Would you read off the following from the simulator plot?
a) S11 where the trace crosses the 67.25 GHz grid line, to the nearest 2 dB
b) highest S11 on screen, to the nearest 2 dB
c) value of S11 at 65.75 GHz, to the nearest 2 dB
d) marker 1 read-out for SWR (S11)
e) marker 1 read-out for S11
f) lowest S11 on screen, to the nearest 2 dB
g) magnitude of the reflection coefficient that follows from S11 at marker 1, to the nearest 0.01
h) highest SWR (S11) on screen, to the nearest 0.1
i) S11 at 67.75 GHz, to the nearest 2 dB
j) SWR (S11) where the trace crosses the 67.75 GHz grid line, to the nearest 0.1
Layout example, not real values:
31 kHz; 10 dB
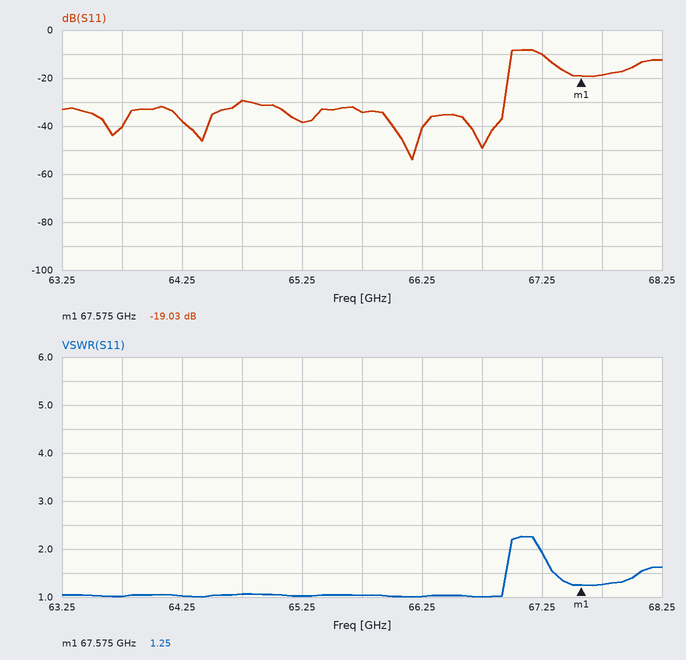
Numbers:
-10 dB; -8 dB; -34 dB; 1.25; -19.03 dB; -54 dB; 0.11; 2.3; -18 dB; 1.3
